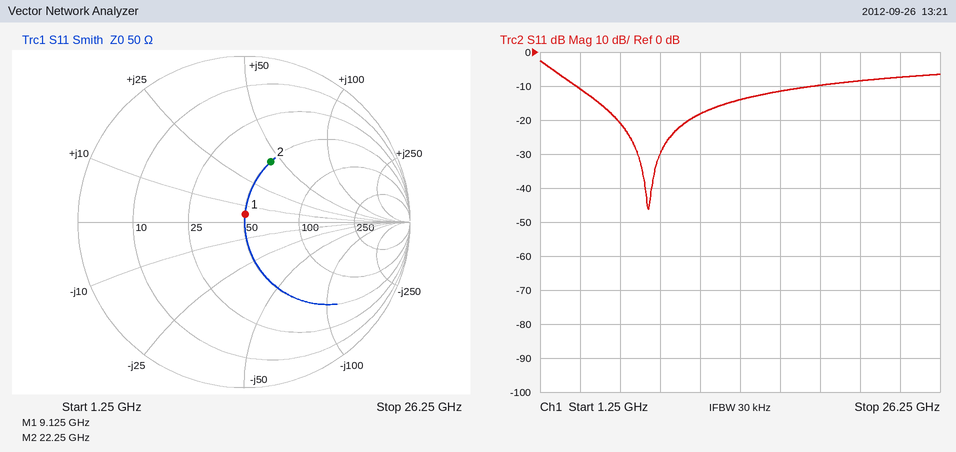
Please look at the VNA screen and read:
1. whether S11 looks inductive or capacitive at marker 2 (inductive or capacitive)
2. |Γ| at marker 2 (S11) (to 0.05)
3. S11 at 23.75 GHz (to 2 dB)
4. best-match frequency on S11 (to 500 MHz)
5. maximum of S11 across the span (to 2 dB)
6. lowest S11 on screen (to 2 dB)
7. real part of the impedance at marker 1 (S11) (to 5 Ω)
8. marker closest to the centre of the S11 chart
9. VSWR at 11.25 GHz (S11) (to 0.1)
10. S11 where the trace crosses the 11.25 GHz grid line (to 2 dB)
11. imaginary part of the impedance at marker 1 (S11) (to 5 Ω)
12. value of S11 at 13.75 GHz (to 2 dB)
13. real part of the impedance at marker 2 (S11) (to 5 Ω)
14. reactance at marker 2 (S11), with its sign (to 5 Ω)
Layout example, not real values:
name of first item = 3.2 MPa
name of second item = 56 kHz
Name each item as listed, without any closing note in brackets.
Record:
whether S11 looks inductive or capacitive at marker 2 = inductive
|Γ| at marker 2 (S11) = 0.40
S11 at 23.75 GHz = -8 dB
best-match frequency on S11 = 8.0 GHz
maximum of S11 across the span = -2 dB
lowest S11 on screen = -46 dB
real part of the impedance at marker 1 (S11) = 50 Ω
marker closest to the centre of the S11 chart = marker 1
VSWR at 11.25 GHz (S11) = 1.3
S11 where the trace crosses the 11.25 GHz grid line = -18 dB
imaginary part of the impedance at marker 1 (S11) = +5 Ω
value of S11 at 13.75 GHz = -14 dB
real part of the impedance at marker 2 (S11) = 50 Ω
reactance at marker 2 (S11), with its sign = +45 Ω
